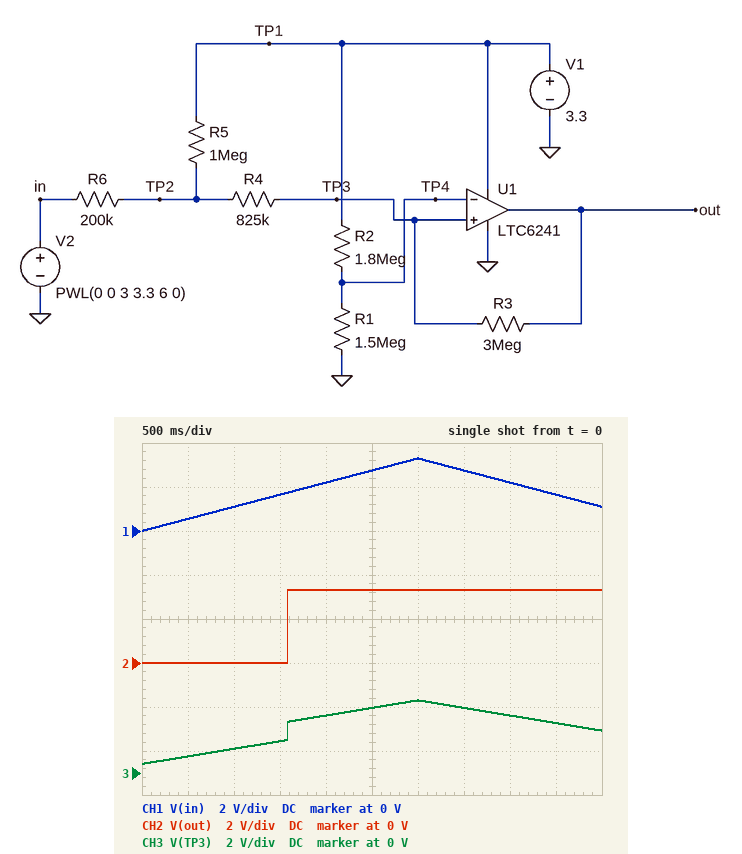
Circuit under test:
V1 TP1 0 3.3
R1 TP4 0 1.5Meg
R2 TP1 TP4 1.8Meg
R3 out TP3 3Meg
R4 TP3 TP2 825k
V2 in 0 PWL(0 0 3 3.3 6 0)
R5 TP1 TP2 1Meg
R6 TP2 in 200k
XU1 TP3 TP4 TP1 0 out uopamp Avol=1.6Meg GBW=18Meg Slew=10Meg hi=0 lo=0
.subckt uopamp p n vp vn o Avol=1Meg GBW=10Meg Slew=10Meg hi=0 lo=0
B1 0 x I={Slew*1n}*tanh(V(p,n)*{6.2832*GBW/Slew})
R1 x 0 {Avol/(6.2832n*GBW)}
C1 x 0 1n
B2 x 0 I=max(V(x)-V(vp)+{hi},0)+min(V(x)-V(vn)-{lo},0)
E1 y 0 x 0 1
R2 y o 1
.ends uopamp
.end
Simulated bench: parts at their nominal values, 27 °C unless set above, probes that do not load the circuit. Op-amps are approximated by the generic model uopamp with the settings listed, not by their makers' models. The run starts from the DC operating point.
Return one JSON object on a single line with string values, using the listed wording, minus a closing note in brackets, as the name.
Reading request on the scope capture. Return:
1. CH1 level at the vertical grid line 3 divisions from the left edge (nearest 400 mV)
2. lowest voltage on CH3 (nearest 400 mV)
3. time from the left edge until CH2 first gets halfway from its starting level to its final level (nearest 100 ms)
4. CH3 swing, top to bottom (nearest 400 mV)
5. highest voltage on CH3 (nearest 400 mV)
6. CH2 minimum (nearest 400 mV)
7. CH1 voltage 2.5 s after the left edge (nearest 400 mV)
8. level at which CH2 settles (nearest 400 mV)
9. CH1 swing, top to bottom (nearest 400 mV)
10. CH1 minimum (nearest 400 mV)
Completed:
{"CH1 level at the vertical grid line 3 divisions from the left edge": "1.6 V", "lowest voltage on CH3": "400 mV", "time from the left edge until CH2 first gets halfway from its starting level to its final level": "1.6 s", "CH3 swing, top to bottom": "2.8 V", "highest voltage on CH3": "3.2 V", "CH2 minimum": "0 V", "CH1 voltage 2.5 s after the left edge": "2.8 V", "level at which CH2 settles": "3.2 V", "CH1 swing, top to bottom": "3.2 V", "CH1 minimum": "0 V"}
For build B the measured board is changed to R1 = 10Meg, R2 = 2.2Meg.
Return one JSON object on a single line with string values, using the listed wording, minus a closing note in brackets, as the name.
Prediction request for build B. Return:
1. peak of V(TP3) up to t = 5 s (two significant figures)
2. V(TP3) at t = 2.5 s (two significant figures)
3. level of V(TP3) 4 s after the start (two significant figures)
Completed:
{"peak of V(TP3) up to t = 5 s": "2.5 V", "V(TP3) at t = 2.5 s": "2.1 V", "level of V(TP3) 4 s after the start": "1.8 V"}
